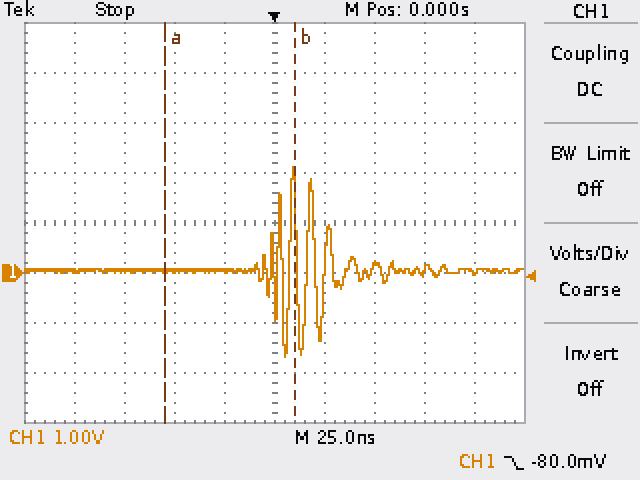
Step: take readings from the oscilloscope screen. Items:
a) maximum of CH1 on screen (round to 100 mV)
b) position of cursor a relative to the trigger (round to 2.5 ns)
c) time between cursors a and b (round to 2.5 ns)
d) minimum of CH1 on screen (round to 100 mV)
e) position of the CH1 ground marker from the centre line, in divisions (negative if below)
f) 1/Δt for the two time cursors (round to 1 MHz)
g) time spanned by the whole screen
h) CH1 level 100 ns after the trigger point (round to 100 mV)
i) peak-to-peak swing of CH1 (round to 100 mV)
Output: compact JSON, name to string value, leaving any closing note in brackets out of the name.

{"maximum of CH1 on screen": "2.1 V", "position of cursor a relative to the trigger": "-55.0 ns", "time between cursors a and b": "65.0 ns", "minimum of CH1 on screen": "-1.7 V", "position of the CH1 ground marker from the centre line, in divisions": "-1.0 div", "1/Δt for the two time cursors": "15 MHz", "time spanned by the whole screen": "250 ns", "CH1 level 100 ns after the trigger point": "0.0 V", "peak-to-peak swing of CH1": "3.8 V"}
